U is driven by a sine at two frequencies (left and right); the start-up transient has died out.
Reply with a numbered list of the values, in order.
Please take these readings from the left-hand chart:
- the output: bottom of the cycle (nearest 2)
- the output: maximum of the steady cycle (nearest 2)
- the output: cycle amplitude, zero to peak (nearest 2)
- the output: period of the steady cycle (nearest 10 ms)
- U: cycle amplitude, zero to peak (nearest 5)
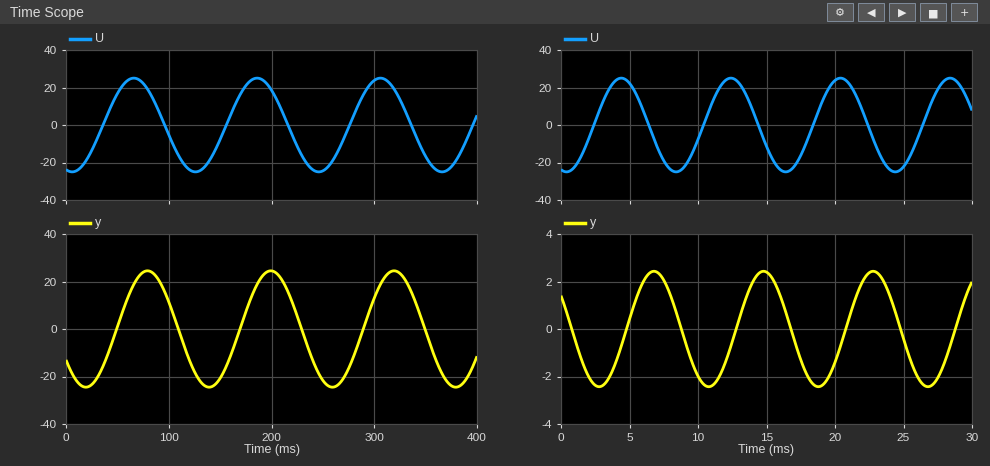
1. -24
2. 24
3. 24
4. 120 ms
5. 25
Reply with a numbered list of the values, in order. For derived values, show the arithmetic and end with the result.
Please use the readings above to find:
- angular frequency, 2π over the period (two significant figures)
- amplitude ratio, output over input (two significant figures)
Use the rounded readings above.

1. 2π / 120 = 0.052 rad/ms
2. 24 / 25 = 0.96
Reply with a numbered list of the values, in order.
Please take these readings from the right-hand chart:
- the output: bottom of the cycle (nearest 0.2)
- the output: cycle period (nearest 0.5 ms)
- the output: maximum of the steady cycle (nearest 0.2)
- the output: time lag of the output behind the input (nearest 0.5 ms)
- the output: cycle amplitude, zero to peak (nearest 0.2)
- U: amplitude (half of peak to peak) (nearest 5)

1. -2.4
2. 8.0 ms
3. 2.4
4. 2.5 ms
5. 2.4
6. 25
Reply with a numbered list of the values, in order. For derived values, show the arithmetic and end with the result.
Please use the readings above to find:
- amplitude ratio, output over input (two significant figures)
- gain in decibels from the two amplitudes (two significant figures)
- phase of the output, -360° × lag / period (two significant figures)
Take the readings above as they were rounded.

1. 2.4 / 25 = 0.096
2. 20 log10(2.4 / 25) = -20 dB
3. -360 × 2.5 / 8 = -110°
